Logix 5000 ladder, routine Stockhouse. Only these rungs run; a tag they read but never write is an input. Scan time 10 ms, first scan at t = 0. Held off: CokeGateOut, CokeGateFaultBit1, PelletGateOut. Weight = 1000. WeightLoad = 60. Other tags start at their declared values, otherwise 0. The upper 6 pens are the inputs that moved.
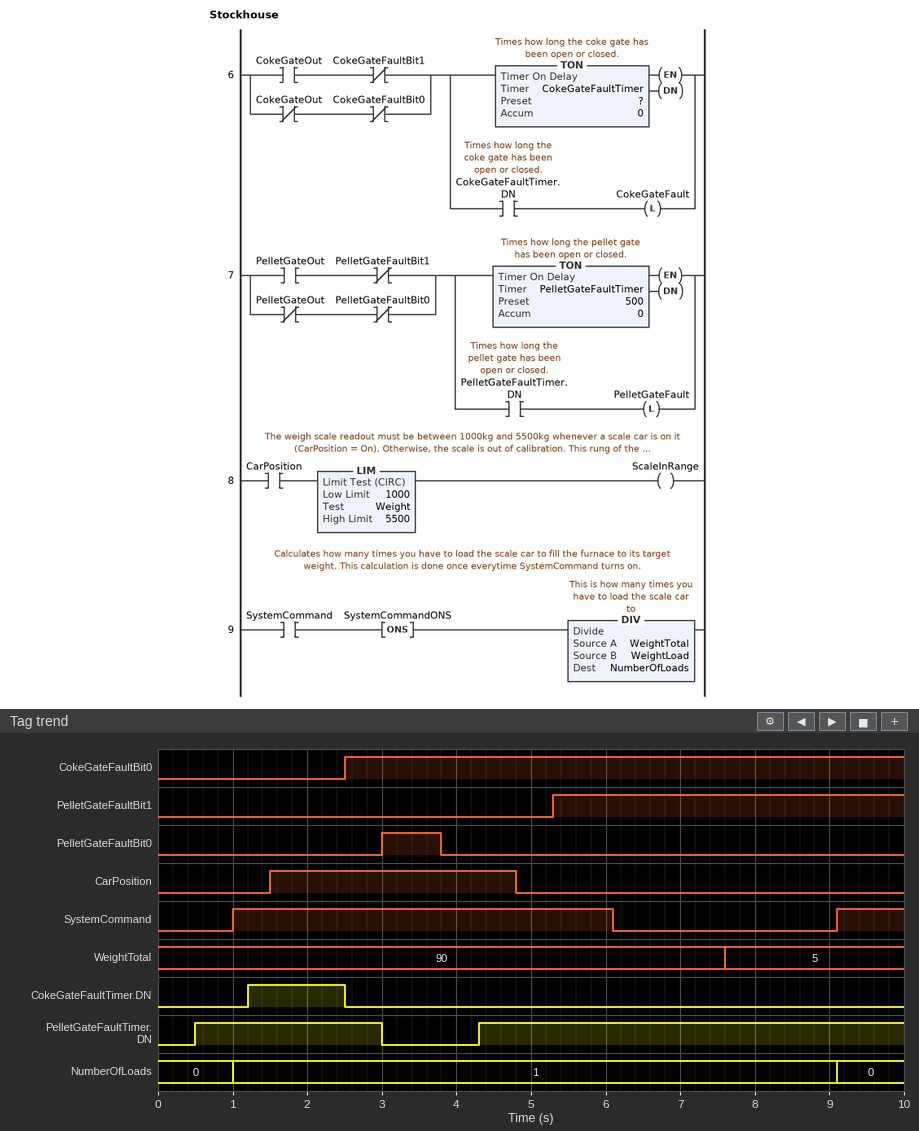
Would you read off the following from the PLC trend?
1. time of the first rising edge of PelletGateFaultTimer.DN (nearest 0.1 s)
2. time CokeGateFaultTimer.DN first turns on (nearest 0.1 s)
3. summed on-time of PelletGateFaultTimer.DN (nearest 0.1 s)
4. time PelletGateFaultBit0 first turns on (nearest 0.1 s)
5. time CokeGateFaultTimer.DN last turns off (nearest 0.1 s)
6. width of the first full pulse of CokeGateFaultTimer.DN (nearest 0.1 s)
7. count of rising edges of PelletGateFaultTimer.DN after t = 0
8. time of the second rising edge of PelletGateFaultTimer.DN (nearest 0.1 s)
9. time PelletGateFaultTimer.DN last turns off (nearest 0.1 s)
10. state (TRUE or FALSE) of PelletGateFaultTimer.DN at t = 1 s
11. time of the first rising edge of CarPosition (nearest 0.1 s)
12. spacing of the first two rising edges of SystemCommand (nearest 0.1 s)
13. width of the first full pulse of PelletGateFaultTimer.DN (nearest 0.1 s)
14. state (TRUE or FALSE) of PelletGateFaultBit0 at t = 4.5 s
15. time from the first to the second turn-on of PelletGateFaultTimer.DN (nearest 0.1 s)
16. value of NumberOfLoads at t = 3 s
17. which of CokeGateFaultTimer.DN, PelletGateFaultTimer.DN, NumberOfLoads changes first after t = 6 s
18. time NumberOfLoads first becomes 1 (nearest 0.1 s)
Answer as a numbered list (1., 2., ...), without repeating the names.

1. 0.5 s
2. 1.2 s
3. 8.2 s
4. 3.0 s
5. 2.5 s
6. 1.3 s
7. 2
8. 4.3 s
9. 3.0 s
10. TRUE
11. 1.5 s
12. 8.1 s
13. 2.5 s
14. FALSE
15. 3.8 s
16. 1
17. NumberOfLoads
18. 1.0 s
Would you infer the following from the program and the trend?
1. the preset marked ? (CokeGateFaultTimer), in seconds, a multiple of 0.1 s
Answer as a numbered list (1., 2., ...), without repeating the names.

1. 1.2 s
